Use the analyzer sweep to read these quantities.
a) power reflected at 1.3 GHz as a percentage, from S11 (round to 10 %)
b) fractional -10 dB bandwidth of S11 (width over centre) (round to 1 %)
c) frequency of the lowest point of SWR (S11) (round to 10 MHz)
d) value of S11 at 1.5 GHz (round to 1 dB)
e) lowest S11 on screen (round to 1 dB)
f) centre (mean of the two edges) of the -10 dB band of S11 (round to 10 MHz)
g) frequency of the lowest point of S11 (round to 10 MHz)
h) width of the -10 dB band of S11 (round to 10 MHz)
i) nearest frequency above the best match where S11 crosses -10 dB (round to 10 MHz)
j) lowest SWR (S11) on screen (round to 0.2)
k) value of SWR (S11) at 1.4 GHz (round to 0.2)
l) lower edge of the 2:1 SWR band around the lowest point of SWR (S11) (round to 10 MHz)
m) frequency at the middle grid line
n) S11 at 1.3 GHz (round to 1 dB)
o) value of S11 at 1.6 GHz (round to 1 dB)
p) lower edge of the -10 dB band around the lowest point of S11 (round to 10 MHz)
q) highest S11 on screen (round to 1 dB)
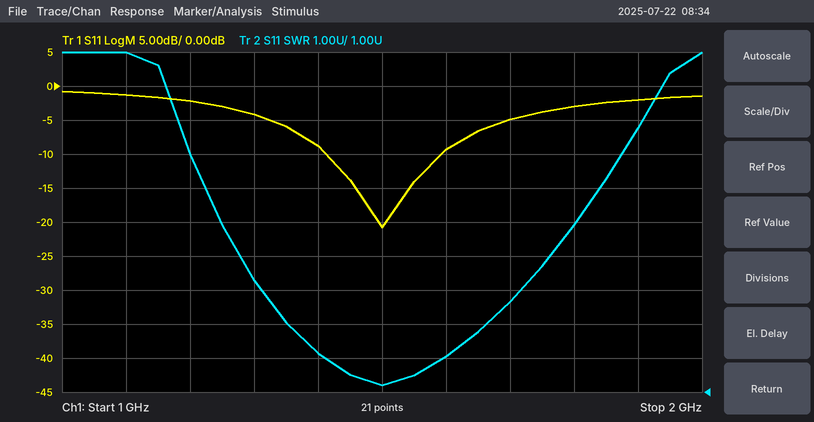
40 %
12 %
1.50 GHz
-21 dB
-21 dB
1.50 GHz
1.50 GHz
180 MHz
1.59 GHz
1.2
2.2
1.41 GHz
1.5 GHz
-4 dB
-9 dB
1.41 GHz
-1 dB
